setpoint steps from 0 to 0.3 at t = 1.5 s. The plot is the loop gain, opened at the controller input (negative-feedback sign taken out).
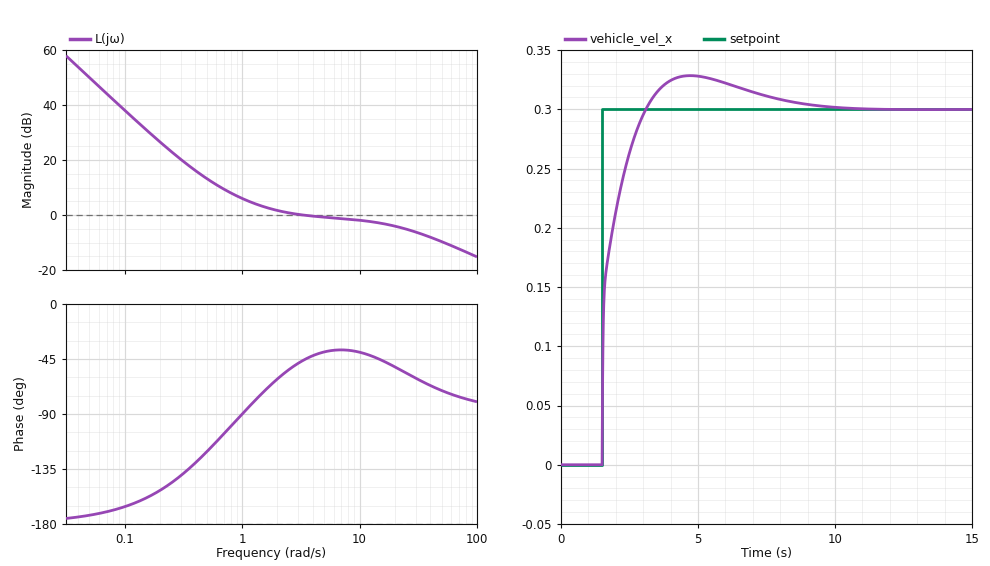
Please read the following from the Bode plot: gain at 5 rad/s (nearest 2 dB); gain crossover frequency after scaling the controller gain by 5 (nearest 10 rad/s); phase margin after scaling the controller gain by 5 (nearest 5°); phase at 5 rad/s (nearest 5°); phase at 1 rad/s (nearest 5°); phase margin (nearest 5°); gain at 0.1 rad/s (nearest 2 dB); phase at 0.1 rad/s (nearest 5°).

0 dB
90 rad/s
100°
-40°
-90°
135°
38 dB
-165°
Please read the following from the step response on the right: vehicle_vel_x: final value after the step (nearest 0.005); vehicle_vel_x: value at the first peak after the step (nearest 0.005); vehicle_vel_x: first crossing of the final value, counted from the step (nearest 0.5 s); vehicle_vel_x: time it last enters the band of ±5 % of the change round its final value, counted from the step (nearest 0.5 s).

0.300
0.330
1.5 s
5.5 s
